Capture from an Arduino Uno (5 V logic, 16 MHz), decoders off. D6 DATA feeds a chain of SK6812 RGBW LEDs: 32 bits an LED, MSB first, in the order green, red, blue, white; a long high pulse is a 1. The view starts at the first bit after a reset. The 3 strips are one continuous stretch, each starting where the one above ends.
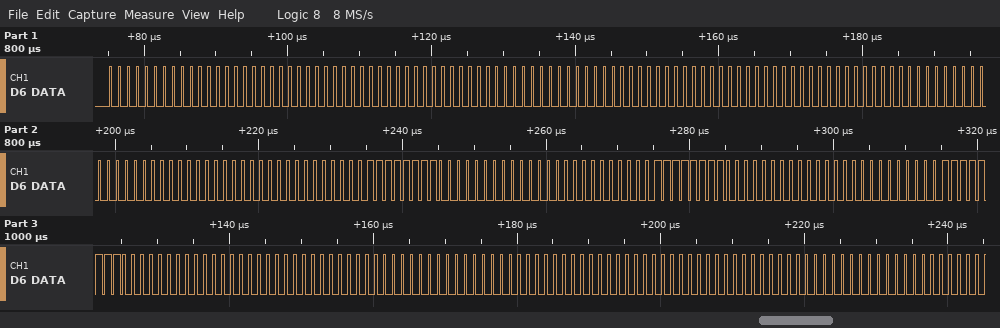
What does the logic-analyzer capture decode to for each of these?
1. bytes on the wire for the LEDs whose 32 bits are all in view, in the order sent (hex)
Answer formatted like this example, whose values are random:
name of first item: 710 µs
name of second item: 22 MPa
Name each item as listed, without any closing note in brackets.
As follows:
bytes on the wire for the LEDs whose 32 bits are all in view, in the order sent: 00 00 00 00 00 00 00 00 00 00 00 00 00 00 00 00 FF 00 00 00 FF 00 00 00 FF 00 00 00 00 00 00 00 00 00 00 00
